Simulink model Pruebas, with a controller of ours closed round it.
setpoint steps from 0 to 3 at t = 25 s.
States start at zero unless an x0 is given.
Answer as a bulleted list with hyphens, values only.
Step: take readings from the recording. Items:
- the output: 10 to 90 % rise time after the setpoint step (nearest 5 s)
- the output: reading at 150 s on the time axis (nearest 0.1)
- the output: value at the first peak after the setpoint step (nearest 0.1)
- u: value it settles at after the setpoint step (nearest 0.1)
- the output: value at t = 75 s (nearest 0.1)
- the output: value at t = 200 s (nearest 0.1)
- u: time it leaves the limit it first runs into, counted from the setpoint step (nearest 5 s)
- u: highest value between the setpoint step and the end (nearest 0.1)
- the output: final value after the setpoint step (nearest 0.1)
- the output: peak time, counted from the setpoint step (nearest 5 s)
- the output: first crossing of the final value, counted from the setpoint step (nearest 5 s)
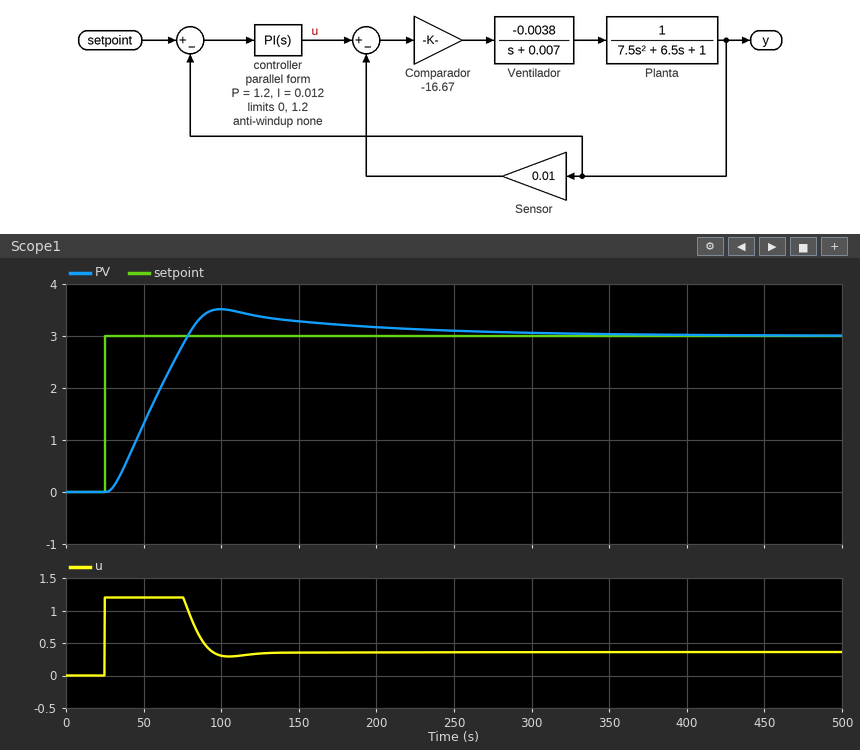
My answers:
- 40 s
- 3.3
- 3.5
- 0.4
- 2.8
- 3.2
- 50 s
- 1.2
- 3.0
- 75 s
- 55 s
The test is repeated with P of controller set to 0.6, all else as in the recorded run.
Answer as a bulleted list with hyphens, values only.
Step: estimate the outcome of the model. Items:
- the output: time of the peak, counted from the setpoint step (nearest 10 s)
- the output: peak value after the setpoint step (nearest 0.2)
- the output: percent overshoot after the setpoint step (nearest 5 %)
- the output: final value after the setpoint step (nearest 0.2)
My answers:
- 90 s
- 3.8
- 25 %
- 3.0
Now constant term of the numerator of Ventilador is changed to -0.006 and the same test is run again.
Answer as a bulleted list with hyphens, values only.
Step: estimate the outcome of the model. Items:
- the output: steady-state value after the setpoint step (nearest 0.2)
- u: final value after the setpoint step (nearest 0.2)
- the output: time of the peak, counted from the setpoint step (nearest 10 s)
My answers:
- 3.0
- 0.2
- 50 s
